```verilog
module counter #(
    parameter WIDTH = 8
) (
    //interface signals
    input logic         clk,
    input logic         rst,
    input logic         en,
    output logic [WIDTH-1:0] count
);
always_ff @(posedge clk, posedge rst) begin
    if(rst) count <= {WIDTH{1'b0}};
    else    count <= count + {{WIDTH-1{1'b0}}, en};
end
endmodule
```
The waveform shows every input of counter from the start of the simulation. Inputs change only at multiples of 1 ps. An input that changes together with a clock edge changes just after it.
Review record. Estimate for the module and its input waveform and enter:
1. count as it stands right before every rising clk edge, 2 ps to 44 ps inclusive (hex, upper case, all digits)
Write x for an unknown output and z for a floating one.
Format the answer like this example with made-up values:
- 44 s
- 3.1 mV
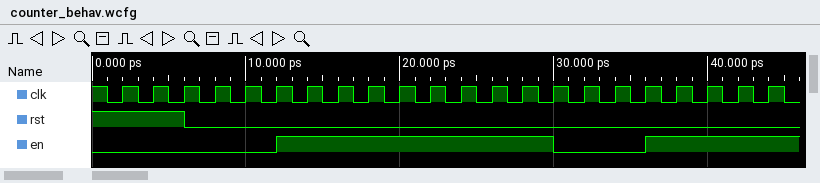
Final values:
- 00, 00, 00, 00, 00, 00, 00, 01, 02, 03, 04, 05, 06, 07, 08, 09, 09, 09, 09, 0A, 0B, 0C
